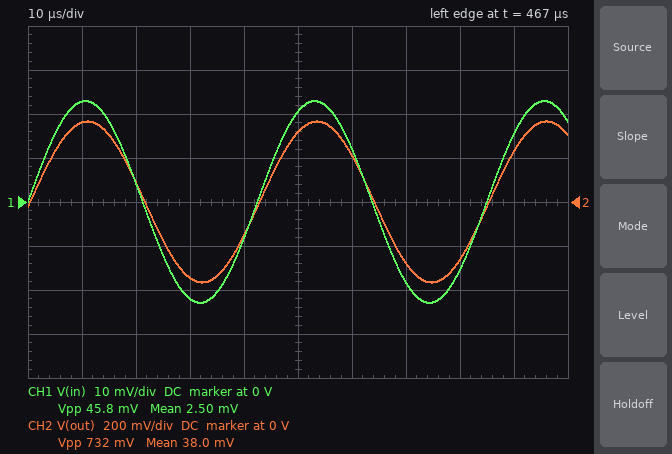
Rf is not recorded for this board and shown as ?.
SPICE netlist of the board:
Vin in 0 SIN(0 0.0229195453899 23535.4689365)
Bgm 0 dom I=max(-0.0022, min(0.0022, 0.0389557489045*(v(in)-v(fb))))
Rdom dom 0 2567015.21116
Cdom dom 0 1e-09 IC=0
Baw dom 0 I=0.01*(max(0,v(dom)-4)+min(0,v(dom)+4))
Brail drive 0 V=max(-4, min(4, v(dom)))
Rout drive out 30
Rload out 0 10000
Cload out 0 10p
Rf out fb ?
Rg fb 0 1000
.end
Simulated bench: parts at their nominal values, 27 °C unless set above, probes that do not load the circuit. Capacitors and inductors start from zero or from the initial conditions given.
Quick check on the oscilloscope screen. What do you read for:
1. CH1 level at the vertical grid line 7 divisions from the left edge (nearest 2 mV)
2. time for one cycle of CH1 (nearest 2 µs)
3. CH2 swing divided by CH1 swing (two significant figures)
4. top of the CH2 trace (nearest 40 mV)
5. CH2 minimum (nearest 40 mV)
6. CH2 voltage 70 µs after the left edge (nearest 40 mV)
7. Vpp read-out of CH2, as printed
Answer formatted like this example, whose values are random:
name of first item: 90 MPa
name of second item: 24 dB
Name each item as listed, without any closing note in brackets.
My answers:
CH1 level at the vertical grid line 7 divisions from the left edge: -18 mV
time for one cycle of CH1: 42 µs
CH2 swing divided by CH1 swing: 16
top of the CH2 trace: 360 mV
CH2 minimum: -360 mV
CH2 voltage 70 µs after the left edge: -280 mV
Vpp read-out of CH2, as printed: 732 mV
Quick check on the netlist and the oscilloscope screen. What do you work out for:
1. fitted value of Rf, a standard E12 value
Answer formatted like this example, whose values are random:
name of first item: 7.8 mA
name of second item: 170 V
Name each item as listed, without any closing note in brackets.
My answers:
fitted value of Rf, a standard E12 value: 15 kΩ
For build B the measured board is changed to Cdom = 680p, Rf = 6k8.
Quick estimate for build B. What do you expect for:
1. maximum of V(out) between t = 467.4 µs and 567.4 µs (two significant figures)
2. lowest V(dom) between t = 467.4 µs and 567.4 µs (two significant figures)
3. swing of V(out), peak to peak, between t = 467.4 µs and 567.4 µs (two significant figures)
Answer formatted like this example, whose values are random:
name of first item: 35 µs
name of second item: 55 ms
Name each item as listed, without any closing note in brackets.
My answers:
maximum of V(out) between t = 467.4 µs and 567.4 µs: 180 mV
lowest V(dom) between t = 467.4 µs and 567.4 µs: -180 mV
swing of V(out), peak to peak, between t = 467.4 µs and 567.4 µs: 360 mV
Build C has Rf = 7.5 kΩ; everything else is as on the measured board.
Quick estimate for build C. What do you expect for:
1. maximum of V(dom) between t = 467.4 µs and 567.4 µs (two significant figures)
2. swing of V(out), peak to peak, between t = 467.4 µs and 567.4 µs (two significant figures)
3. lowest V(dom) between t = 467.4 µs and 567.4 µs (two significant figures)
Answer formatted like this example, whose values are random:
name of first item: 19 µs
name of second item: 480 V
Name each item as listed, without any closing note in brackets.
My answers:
maximum of V(dom) between t = 467.4 µs and 567.4 µs: 200 mV
swing of V(out), peak to peak, between t = 467.4 µs and 567.4 µs: 390 mV
lowest V(dom) between t = 467.4 µs and 567.4 µs: -200 mV
